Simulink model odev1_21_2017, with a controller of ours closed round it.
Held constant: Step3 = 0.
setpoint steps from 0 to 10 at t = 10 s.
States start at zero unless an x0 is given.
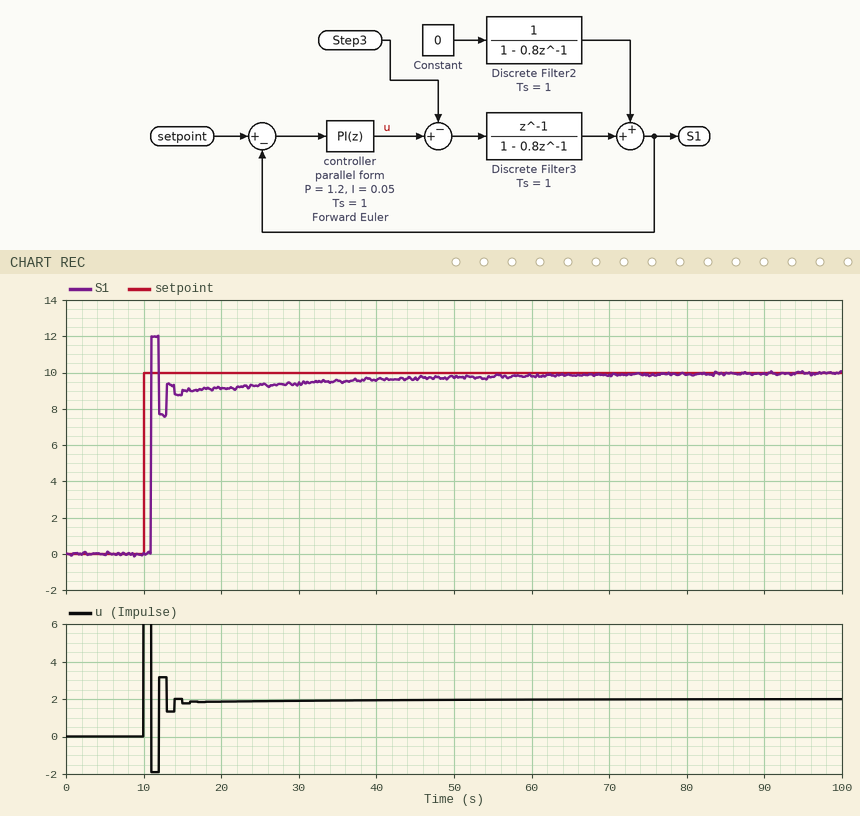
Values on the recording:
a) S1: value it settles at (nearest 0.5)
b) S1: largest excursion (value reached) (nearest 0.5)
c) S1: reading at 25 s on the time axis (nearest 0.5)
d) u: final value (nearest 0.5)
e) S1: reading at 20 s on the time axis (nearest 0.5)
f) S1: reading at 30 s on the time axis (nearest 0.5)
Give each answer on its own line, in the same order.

10.0
12.0
9.5
2.0
9.0
9.5
